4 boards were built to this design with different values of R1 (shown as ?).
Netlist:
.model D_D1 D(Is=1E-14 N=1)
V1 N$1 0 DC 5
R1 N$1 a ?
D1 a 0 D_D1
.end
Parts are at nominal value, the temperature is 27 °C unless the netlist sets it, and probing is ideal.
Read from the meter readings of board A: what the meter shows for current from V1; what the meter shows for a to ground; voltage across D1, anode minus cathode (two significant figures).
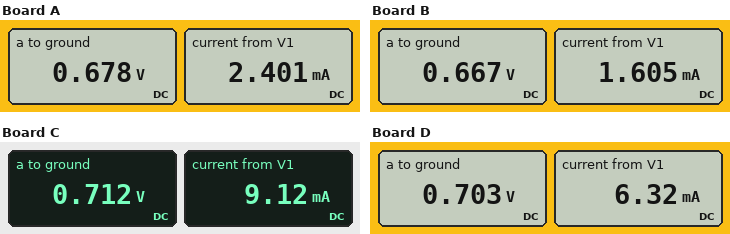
2.401 mA
0.678 V
680 mV
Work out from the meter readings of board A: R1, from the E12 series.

1.8 kΩ
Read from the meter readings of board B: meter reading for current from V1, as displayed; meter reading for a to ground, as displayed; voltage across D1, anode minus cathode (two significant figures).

1.605 mA
0.667 V
670 mV
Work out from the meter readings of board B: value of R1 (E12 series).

2.7 kΩ
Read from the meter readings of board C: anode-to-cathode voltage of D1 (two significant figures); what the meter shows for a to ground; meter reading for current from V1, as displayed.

710 mV
0.712 V
9.12 mA
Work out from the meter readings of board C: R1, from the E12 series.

470 Ω
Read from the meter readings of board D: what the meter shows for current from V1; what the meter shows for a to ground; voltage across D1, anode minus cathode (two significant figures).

6.32 mA
0.703 V
700 mV
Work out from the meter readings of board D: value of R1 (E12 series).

680 Ω
